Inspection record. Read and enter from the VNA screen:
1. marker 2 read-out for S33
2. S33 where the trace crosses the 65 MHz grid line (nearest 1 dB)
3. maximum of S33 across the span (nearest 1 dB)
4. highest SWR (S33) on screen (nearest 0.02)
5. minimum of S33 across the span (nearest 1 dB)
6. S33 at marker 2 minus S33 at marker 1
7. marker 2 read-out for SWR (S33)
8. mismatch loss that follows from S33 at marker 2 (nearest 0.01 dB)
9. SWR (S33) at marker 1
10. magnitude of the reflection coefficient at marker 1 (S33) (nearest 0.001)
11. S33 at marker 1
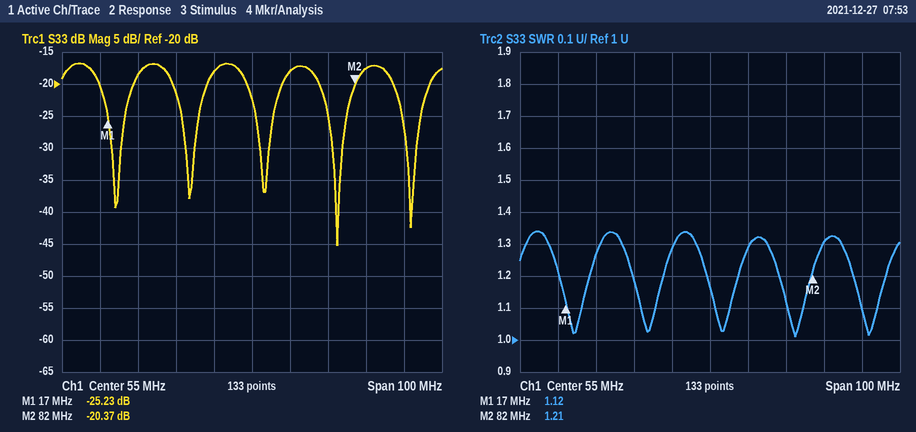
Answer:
-20.37 dB
-18 dB
-17 dB
1.34
-45 dB
4.86 dB
1.21
0.04 dB
1.12
0.055
-25.23 dB
